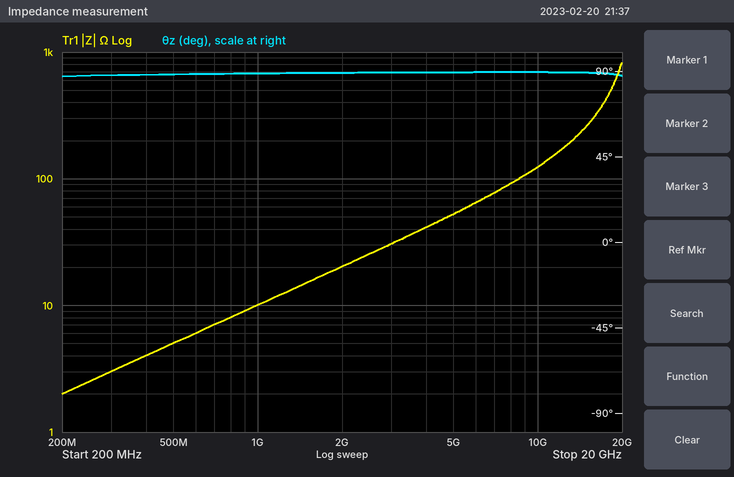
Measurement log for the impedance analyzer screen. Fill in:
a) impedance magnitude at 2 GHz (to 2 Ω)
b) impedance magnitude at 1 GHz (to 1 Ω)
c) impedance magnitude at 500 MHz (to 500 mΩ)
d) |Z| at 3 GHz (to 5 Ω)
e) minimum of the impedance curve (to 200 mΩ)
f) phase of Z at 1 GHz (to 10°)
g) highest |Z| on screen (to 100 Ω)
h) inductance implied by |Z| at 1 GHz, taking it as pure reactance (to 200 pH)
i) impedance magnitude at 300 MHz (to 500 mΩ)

20 Ω
10 Ω
5.0 Ω
30 Ω
2.0 Ω
90°
800 Ω
1.6 nH
3.0 Ω
